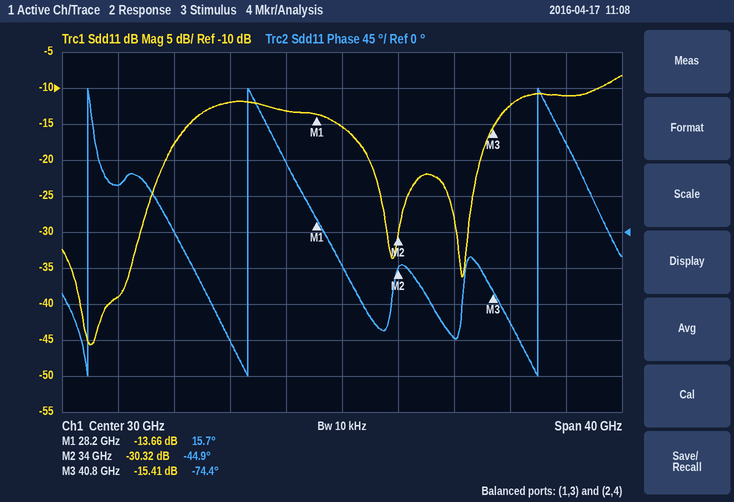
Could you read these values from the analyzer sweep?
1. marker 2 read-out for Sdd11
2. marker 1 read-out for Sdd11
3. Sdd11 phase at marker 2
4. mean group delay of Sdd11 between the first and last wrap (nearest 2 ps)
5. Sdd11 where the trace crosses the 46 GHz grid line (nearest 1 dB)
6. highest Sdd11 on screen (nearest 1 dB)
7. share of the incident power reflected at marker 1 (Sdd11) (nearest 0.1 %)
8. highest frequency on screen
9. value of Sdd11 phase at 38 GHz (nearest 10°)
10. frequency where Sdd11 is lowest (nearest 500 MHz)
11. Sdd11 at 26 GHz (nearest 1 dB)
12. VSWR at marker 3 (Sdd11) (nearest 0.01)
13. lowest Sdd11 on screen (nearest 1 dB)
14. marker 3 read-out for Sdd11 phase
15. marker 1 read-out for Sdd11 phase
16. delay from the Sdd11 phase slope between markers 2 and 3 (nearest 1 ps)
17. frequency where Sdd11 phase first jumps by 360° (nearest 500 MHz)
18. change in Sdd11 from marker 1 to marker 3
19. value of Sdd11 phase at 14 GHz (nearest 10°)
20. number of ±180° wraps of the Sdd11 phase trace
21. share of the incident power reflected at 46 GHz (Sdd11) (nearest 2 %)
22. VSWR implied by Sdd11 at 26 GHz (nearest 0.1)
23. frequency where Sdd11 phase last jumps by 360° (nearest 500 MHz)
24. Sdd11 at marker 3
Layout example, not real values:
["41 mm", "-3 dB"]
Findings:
["-30.32 dB", "-13.66 dB", "-44.9°", "62 ps", "-11 dB", "-8 dB", "4.3 %", "50 GHz", "-130°", "12.0 GHz", "-13 dB", "1.41", "-46 dB", "-74.4°", "15.7°", "12 ps", "12.0 GHz", "-1.75 dB", "60°", "3", "8 %", "1.6", "44.0 GHz", "-15.41 dB"]
